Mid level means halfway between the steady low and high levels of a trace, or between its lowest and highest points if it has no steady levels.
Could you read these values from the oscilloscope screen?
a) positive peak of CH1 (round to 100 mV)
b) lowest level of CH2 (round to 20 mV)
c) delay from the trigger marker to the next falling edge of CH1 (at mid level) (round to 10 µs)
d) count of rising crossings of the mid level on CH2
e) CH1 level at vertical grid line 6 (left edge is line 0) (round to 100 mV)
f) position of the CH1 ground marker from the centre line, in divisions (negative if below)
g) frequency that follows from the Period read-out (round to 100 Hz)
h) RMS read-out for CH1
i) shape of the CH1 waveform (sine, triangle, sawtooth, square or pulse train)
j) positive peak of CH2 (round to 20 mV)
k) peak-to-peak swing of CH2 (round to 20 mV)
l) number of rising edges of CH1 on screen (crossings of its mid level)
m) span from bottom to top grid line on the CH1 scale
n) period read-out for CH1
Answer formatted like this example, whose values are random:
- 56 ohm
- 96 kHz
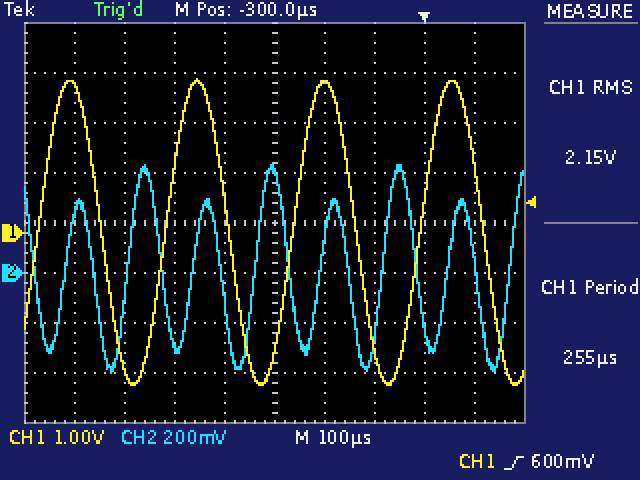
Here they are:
- 3.1 V
- -400 mV
- 120 µs
- 8
- 3.0 V
- -0.2 div
- 3.9 kHz
- 2.15 V
- sine
- 440 mV
- 840 mV
- 4
- 8 V
- 255 µs
